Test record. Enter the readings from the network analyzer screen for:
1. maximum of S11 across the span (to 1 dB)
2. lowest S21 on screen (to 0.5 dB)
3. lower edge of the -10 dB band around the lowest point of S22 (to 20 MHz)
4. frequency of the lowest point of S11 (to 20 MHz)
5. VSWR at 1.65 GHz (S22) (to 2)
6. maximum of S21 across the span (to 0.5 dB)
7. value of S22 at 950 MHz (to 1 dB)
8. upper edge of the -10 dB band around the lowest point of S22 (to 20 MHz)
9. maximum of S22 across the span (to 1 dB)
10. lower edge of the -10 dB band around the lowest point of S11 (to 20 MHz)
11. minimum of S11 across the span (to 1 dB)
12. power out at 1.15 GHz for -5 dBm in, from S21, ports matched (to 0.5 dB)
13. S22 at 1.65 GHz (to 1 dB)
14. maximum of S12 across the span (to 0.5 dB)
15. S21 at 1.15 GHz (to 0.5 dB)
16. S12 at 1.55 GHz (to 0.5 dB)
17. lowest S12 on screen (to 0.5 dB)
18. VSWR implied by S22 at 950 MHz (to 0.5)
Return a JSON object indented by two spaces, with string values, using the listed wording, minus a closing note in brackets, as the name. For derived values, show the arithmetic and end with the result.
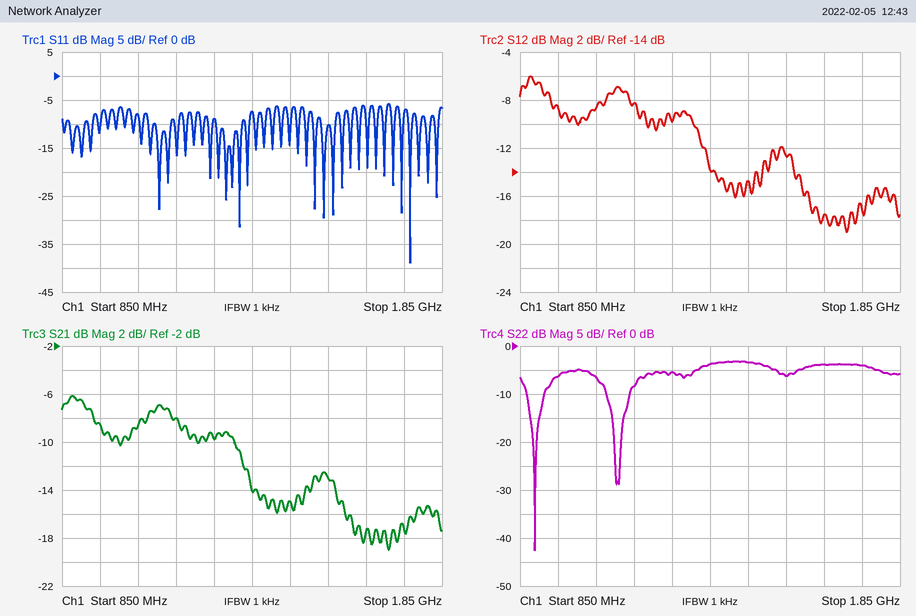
{
  "maximum of S11 across the span": "-6 dB",
  "lowest S21 on screen": "-19.0 dB",
  "lower edge of the -10 dB band around the lowest point of S22": "860 MHz",
  "frequency of the lowest point of S11": "1.76 GHz",
  "VSWR at 1.65 GHz (S22)": "|Γ| = 10^(-4/20) = 0.6310; VSWR = (1 + 0.6310)/(1 − 0.6310) ≈ 4",
  "maximum of S21 across the span": "-6.0 dB",
  "value of S22 at 950 MHz": "-6 dB",
  "upper edge of the -10 dB band around the lowest point of S22": "920 MHz",
  "maximum of S22 across the span": "-3 dB",
  "lower edge of the -10 dB band around the lowest point of S11": "1.76 GHz",
  "minimum of S11 across the span": "-39 dB",
  "power out at 1.15 GHz for -5 dBm in, from S21, ports matched": "-5 dBm + (-8.0 dB) = -13.0 dBm",
  "S22 at 1.65 GHz": "-4 dB",
  "maximum of S12 across the span": "-6.0 dB",
  "S21 at 1.15 GHz": "-8.0 dB",
  "S12 at 1.55 GHz": "-12.5 dB",
  "lowest S12 on screen": "-19.0 dB",
  "VSWR implied by S22 at 950 MHz": "|Γ| = 10^(-6/20) = 0.5012; VSWR = (1 + 0.5012)/(1 − 0.5012) ≈ 3.0"
}
